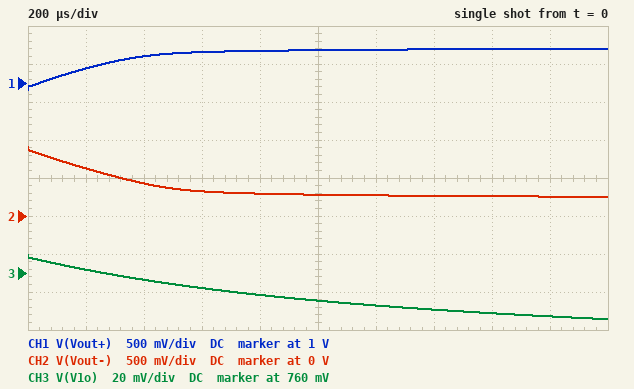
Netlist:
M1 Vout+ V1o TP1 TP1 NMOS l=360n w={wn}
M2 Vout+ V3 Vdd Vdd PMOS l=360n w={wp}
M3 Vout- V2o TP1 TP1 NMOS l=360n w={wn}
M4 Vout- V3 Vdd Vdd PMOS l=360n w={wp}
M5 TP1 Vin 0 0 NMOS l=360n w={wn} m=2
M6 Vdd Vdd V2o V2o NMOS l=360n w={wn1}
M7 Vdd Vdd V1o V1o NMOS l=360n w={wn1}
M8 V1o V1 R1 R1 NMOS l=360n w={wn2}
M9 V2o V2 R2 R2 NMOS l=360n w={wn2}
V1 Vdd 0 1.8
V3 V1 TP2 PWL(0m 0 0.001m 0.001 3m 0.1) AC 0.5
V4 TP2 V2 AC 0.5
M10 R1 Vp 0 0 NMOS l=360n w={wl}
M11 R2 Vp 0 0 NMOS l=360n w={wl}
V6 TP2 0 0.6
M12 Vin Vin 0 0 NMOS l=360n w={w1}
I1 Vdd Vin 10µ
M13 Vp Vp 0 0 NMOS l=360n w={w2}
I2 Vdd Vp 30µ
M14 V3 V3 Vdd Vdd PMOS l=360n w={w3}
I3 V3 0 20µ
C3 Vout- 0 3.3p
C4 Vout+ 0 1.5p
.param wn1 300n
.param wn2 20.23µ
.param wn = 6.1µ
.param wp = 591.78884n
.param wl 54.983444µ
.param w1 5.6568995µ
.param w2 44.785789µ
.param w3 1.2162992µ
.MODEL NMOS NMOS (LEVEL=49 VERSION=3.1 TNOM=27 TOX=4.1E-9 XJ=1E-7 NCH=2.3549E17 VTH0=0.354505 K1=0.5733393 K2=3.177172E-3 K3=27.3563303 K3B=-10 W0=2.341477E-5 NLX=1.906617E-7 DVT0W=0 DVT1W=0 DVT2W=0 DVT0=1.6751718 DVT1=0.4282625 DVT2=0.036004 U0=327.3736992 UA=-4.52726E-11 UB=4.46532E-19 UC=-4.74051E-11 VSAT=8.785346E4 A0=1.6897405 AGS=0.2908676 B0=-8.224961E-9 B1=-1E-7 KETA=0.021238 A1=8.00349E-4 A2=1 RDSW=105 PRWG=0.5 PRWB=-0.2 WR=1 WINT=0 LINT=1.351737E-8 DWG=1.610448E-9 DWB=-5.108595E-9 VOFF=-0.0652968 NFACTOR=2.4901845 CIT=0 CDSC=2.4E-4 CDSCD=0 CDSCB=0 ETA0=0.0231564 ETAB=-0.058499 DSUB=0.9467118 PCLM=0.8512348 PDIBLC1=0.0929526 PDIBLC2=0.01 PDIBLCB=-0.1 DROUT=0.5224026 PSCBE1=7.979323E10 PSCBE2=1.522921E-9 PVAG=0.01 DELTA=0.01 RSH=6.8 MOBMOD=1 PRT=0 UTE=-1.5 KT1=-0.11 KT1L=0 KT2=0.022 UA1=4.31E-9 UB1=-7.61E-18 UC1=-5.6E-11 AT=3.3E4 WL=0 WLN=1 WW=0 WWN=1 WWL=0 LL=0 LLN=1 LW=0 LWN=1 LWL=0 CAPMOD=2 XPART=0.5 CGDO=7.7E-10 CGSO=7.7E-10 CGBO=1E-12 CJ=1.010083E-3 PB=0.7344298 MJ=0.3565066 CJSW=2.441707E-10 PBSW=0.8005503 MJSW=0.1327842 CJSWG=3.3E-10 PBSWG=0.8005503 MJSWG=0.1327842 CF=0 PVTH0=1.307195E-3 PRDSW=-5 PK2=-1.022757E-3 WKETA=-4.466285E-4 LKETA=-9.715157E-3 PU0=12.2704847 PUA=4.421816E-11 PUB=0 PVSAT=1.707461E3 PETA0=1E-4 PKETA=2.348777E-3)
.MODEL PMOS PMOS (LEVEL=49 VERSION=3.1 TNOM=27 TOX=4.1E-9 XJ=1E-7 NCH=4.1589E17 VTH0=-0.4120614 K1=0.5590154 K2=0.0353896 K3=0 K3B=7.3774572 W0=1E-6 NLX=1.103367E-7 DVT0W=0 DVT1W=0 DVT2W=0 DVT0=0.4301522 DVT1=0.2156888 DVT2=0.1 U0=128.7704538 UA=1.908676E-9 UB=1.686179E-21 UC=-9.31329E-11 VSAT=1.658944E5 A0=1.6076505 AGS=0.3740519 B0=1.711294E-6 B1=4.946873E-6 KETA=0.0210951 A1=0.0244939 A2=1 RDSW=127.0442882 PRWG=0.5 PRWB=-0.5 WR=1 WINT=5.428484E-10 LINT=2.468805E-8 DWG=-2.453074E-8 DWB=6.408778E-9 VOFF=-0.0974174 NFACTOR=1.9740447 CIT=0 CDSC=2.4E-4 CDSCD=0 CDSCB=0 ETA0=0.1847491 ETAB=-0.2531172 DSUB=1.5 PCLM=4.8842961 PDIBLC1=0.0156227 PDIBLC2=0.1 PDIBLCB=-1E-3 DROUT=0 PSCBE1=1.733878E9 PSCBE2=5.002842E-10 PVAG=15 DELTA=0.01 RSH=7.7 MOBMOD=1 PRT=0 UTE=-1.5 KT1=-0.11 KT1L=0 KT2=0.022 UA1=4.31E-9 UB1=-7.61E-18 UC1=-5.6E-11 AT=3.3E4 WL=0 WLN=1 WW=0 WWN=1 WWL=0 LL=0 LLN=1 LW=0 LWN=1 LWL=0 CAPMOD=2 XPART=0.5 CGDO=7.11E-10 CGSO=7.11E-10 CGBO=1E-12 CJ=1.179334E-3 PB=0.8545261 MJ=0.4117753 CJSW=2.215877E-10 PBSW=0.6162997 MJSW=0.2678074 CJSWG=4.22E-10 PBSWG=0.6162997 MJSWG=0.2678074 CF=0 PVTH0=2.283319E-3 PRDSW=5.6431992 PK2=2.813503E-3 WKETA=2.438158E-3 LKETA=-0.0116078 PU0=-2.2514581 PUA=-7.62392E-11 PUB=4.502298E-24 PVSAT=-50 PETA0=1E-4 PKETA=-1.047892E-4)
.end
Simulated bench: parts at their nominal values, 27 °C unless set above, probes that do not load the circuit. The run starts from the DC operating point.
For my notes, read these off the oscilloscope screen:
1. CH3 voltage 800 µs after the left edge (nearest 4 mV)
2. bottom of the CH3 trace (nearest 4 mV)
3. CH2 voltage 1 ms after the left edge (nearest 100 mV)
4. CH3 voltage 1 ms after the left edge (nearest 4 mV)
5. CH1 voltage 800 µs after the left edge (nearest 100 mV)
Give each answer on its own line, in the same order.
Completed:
748 mV
736 mV
300 mV
744 mV
1.4 V
